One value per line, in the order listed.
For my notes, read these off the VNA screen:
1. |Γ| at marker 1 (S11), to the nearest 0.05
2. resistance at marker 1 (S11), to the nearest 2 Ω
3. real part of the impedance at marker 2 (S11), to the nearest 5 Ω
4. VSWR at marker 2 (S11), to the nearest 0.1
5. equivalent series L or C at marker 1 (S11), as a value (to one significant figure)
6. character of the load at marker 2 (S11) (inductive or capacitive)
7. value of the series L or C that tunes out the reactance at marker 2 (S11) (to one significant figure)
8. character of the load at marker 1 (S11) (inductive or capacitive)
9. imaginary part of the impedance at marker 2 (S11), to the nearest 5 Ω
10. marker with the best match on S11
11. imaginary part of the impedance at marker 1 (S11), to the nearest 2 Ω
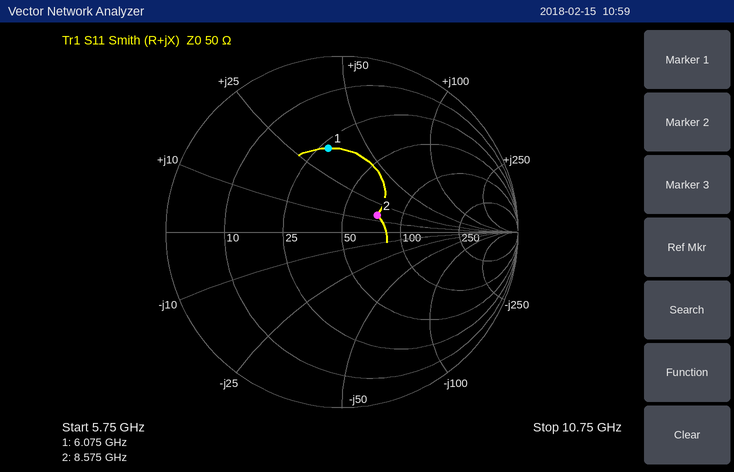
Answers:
0.50
28 Ω
75 Ω
1.6
900 pH
inductive
1 pF
inductive
+15 Ω
marker 2
+34 Ω
